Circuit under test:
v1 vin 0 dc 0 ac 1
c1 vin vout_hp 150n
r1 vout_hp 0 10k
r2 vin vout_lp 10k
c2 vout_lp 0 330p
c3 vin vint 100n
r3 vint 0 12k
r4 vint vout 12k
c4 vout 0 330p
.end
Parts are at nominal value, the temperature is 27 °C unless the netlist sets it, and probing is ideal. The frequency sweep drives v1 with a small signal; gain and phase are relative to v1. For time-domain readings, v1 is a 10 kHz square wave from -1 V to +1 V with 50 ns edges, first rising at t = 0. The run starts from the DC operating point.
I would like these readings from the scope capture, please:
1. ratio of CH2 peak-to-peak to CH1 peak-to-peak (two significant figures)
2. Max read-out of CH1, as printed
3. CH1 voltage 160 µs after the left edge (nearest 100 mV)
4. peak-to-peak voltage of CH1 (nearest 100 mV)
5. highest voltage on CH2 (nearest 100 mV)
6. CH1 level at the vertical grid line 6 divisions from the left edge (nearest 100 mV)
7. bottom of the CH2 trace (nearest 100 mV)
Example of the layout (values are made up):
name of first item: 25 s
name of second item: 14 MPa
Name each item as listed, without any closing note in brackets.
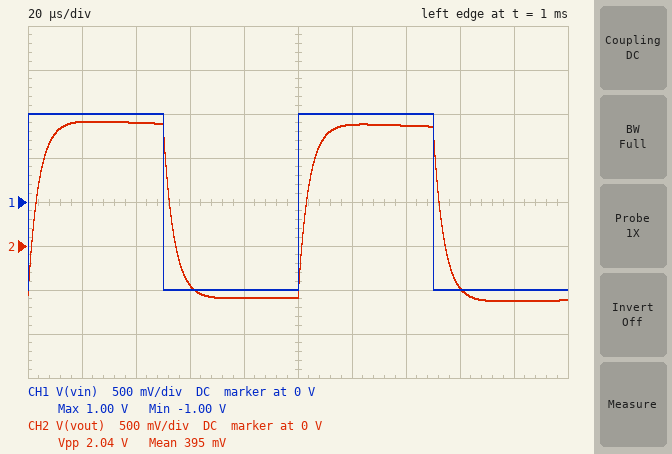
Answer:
ratio of CH2 peak-to-peak to CH1 peak-to-peak: 1.0
Max read-out of CH1, as printed: 1.00 V
CH1 voltage 160 µs after the left edge: -1.0 V
peak-to-peak voltage of CH1: 2.0 V
highest voltage on CH2: 1.4 V
CH1 level at the vertical grid line 6 divisions from the left edge: 1.0 V
bottom of the CH2 trace: -600 mV
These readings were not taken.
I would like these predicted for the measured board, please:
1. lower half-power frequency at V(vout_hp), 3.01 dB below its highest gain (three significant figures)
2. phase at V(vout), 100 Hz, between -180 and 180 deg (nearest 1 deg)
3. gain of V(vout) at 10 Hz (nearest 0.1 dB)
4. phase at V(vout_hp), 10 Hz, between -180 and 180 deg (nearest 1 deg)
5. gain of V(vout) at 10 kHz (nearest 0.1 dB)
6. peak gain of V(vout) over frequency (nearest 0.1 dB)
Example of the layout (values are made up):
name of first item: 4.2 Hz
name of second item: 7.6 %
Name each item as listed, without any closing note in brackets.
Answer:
lower half-power frequency at V(vout_hp), 3.01 dB below its highest gain: 106 Hz
phase at V(vout), 100 Hz, between -180 and 180 deg: 53 deg
gain of V(vout) at 10 Hz: -22.5 dB
phase at V(vout_hp), 10 Hz, between -180 and 180 deg: 85 deg
gain of V(vout) at 10 kHz: -0.3 dB
peak gain of V(vout) over frequency: -0.1 dB
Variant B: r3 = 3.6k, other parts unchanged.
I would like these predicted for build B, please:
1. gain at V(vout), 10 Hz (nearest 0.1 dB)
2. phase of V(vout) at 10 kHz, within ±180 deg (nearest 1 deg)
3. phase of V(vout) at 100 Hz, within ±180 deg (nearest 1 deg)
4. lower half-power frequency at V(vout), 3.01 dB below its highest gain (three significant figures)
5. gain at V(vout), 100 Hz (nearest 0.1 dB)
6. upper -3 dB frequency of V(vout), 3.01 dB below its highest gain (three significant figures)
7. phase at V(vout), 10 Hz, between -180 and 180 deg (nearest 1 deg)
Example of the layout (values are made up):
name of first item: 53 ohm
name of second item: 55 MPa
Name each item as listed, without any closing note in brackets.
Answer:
gain at V(vout), 10 Hz: -32.9 dB
phase of V(vout) at 10 kHz, within ±180 deg: -11 deg
phase of V(vout) at 100 Hz, within ±180 deg: 77 deg
lower half-power frequency at V(vout), 3.01 dB below its highest gain: 431 Hz
gain at V(vout), 100 Hz: -13.1 dB
upper -3 dB frequency of V(vout), 3.01 dB below its highest gain: 41.2 kHz
phase at V(vout), 10 Hz, between -180 and 180 deg: 89 deg
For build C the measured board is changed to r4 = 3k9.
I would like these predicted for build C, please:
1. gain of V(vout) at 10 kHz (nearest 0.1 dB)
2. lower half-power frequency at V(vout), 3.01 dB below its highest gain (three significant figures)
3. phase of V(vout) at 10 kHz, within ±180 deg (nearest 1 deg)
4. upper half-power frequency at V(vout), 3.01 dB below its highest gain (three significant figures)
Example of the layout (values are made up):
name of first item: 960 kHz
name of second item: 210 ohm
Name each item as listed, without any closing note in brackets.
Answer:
gain of V(vout) at 10 kHz: -0.1 dB
lower half-power frequency at V(vout), 3.01 dB below its highest gain: 132 Hz
phase of V(vout) at 10 kHz, within ±180 deg: -4 deg
upper half-power frequency at V(vout), 3.01 dB below its highest gain: 124 kHz
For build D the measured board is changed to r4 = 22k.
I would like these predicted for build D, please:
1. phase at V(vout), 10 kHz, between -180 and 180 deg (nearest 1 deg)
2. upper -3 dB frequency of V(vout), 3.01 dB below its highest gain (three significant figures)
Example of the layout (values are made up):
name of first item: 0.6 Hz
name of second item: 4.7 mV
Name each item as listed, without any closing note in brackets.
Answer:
phase at V(vout), 10 kHz, between -180 and 180 deg: -24 deg
upper -3 dB frequency of V(vout), 3.01 dB below its highest gain: 22.3 kHz
